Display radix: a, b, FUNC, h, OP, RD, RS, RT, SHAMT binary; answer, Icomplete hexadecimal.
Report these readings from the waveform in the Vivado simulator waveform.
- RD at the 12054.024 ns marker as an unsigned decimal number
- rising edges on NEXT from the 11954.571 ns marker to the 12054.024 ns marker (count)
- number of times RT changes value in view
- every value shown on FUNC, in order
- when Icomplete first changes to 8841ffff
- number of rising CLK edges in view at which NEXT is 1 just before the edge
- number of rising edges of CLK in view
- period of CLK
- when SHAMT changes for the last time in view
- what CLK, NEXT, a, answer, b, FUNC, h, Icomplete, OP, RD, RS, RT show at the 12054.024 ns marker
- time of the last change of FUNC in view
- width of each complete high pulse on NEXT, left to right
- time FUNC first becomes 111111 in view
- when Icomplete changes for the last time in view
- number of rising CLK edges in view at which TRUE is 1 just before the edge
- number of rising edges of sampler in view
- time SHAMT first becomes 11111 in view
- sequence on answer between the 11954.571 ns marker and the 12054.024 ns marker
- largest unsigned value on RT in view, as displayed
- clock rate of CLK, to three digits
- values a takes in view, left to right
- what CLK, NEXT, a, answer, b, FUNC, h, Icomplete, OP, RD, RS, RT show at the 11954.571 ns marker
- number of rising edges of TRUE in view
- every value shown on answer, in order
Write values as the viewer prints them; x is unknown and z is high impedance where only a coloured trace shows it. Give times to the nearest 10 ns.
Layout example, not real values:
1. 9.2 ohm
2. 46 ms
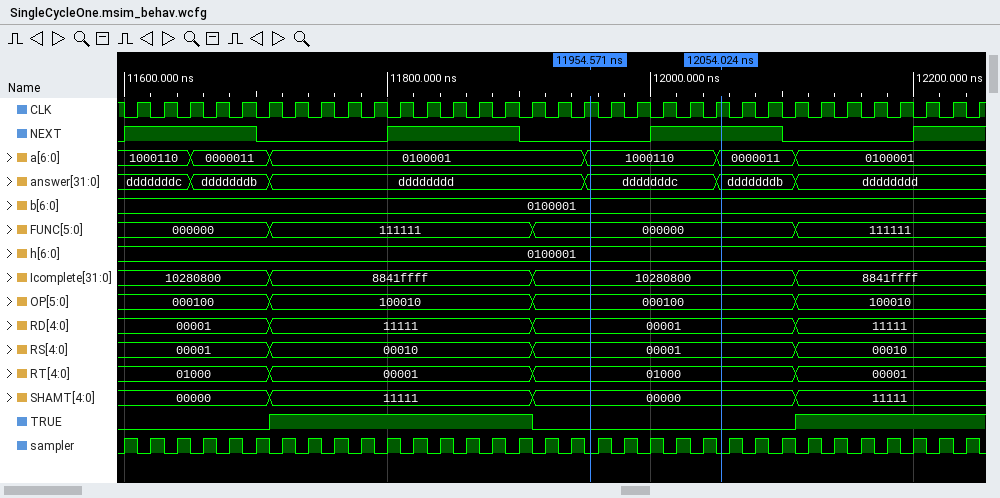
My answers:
1. 1
2. 1
3. 3
4. 000000, 111111, 000000, 111111
5. 11710 ns
6. 18
7. 33
8. 20 ns
9. 12110 ns
10. CLK=1, NEXT=1, a=0000011, answer=dddddddb, b=0100001, FUNC=000000, h=0100001, Icomplete=10280800, OP=000100, RD=00001, RS=00001, RT=01000
11. 12110 ns
12. 100 ns, 100 ns, 100 ns
13. 11710 ns
14. 12110 ns
15. 17
16. 33
17. 11710 ns
18. dddddddc, dddddddb
19. 01000
20. 50.0 MHz
21. 1000110, 0000011, 0100001, 1000110, 0000011, 0100001
22. CLK=1, NEXT=0, a=1000110, answer=dddddddc, b=0100001, FUNC=000000, h=0100001, Icomplete=10280800, OP=000100, RD=00001, RS=00001, RT=01000
23. 2
24. dddddddc, dddddddb, dddddddd, dddddddc, dddddddb, dddddddd
